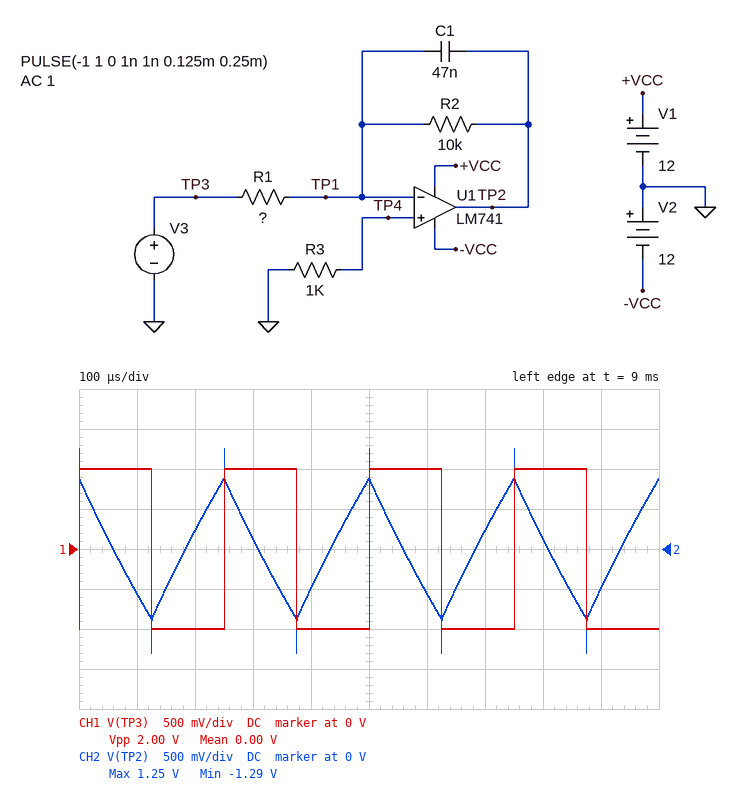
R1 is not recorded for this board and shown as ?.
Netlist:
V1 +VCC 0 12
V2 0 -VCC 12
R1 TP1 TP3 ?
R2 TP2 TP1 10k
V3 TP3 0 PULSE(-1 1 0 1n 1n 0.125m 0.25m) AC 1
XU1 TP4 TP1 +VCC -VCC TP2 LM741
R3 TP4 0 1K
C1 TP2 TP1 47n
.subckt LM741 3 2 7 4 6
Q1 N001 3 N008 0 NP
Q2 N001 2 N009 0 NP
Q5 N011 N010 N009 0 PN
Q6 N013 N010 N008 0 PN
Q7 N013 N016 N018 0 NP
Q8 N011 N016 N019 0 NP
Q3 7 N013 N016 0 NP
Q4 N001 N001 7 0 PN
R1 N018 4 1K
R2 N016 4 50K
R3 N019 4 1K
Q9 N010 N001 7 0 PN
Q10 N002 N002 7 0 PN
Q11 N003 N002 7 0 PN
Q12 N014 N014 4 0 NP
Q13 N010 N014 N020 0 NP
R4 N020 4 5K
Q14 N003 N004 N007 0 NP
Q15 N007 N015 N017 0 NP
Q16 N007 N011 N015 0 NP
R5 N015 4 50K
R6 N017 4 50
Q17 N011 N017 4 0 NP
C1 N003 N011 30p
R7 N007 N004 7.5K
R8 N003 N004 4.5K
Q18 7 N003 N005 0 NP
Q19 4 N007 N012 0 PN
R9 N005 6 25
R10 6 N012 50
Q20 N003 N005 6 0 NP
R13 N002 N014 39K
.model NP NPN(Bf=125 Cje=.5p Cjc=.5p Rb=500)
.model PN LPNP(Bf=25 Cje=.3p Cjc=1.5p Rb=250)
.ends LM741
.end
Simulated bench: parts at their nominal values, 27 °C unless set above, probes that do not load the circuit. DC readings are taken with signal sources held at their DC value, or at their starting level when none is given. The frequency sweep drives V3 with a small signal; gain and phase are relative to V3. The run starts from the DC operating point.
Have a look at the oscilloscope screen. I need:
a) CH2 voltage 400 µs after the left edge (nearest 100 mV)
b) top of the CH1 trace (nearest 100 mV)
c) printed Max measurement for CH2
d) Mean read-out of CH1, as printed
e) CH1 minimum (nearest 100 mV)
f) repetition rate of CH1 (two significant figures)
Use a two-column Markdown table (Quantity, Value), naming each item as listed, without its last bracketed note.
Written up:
| Quantity | Value |
|---|---|
| CH2 voltage 400 µs after the left edge | -500 mV |
| top of the CH1 trace | 1.0 V |
| printed Max measurement for CH2 | 1.25 V |
| Mean read-out of CH1, as printed | 0.00 V |
| CH1 minimum | -1.0 V |
| repetition rate of CH1 | 4.0 kHz |
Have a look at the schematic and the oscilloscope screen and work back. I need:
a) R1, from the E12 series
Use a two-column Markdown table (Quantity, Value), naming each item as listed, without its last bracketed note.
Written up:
| Quantity | Value |
|---|---|
| R1, from the E12 series | 1.5 kΩ |
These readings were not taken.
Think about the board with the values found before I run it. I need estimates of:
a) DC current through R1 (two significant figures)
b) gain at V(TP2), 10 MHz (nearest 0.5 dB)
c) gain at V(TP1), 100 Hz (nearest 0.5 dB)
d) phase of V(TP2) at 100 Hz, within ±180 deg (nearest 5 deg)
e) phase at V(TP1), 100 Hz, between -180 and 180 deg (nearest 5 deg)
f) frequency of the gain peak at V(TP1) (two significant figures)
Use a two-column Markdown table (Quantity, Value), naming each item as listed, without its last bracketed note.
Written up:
| Quantity | Value |
|---|---|
| DC current through R1 | 670 µA |
| gain at V(TP2), 10 MHz | -27.0 dB |
| gain at V(TP1), 100 Hz | -63.0 dB |
| phase of V(TP2) at 100 Hz, within ±180 deg | 165 deg |
| phase at V(TP1), 100 Hz, between -180 and 180 deg | 75 deg |
| frequency of the gain peak at V(TP1) | 920 MHz |
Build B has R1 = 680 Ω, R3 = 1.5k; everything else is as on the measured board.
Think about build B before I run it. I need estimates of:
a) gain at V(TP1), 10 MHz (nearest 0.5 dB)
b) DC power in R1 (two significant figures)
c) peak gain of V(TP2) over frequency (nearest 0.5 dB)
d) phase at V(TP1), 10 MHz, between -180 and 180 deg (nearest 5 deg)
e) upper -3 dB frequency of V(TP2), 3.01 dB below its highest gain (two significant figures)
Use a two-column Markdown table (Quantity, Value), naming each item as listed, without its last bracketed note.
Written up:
| Quantity | Value |
|---|---|
| gain at V(TP1), 10 MHz | -23.0 dB |
| DC power in R1 | 880 µW |
| peak gain of V(TP2) over frequency | -20.0 dB |
| phase at V(TP1), 10 MHz, between -180 and 180 deg | 0 deg |
| upper -3 dB frequency of V(TP2), 3.01 dB below its highest gain | 4.2 GHz |
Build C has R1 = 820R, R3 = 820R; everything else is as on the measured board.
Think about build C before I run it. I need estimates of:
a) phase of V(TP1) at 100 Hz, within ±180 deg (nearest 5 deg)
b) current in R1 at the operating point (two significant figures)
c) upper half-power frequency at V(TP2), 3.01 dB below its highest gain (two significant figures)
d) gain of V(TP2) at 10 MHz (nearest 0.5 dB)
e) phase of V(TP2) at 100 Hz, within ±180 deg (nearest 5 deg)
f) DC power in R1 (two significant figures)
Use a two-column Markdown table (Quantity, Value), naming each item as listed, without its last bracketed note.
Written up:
| Quantity | Value |
|---|---|
| phase of V(TP1) at 100 Hz, within ±180 deg | 0 deg |
| current in R1 at the operating point | 1.1 mA |
| upper half-power frequency at V(TP2), 3.01 dB below its highest gain | 4.1 GHz |
| gain of V(TP2) at 10 MHz | -24.5 dB |
| phase of V(TP2) at 100 Hz, within ±180 deg | 15 deg |
| DC power in R1 | 1.0 mW |
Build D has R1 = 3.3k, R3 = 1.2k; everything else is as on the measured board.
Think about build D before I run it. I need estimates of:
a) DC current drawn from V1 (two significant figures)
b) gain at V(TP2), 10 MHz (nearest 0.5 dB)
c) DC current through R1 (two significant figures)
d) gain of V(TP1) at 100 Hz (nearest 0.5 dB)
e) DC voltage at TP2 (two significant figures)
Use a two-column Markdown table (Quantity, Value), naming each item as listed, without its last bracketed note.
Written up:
| Quantity | Value |
|---|---|
| DC current drawn from V1 | 1.5 mA |
| gain at V(TP2), 10 MHz | -29.0 dB |
| DC current through R1 | 300 µA |
| gain of V(TP1) at 100 Hz | -70.0 dB |
| DC voltage at TP2 | 3.0 V |
